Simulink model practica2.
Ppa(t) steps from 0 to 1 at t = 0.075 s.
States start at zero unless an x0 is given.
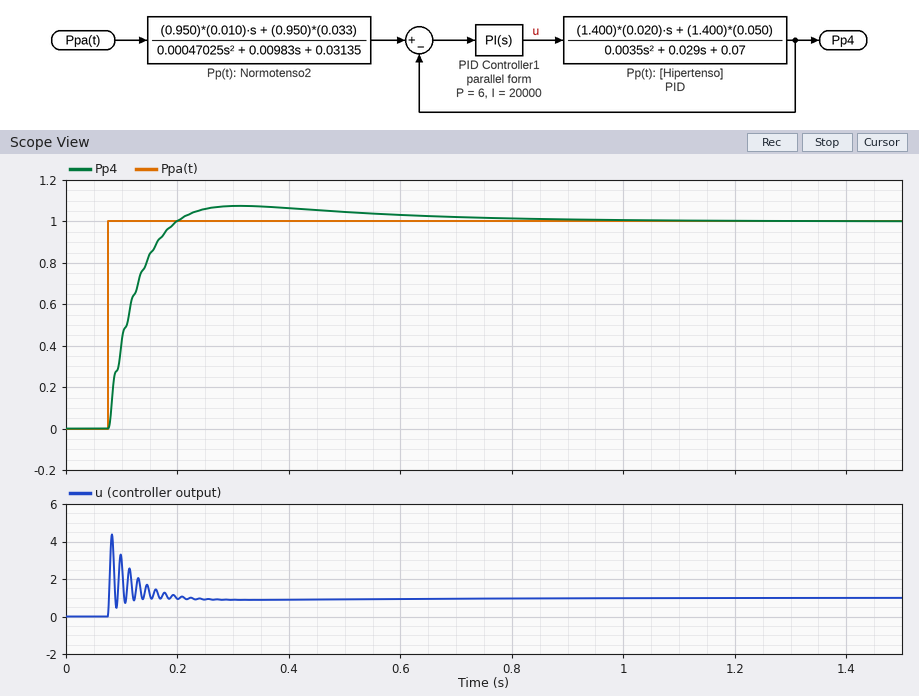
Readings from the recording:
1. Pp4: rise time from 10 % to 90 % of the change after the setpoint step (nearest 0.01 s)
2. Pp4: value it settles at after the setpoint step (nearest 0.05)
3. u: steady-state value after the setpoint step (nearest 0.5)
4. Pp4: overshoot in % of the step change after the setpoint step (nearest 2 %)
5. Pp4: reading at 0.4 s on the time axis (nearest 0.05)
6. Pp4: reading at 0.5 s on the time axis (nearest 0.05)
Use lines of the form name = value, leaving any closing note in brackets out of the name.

Pp4: rise time from 10 % to 90 % of the change after the setpoint step = 0.08 s
Pp4: value it settles at after the setpoint step = 1.00
u: steady-state value after the setpoint step = 1.0
Pp4: overshoot in % of the step change after the setpoint step = 8 %
Pp4: reading at 0.4 s on the time axis = 1.05
Pp4: reading at 0.5 s on the time axis = 1.05
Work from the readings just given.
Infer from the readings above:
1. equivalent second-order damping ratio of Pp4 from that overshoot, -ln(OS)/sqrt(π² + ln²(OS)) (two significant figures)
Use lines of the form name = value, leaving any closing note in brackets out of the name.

equivalent second-order damping ratio of Pp4 from that overshoot, -ln(OS)/sqrt(π² + ln²(OS)) = 0.63
